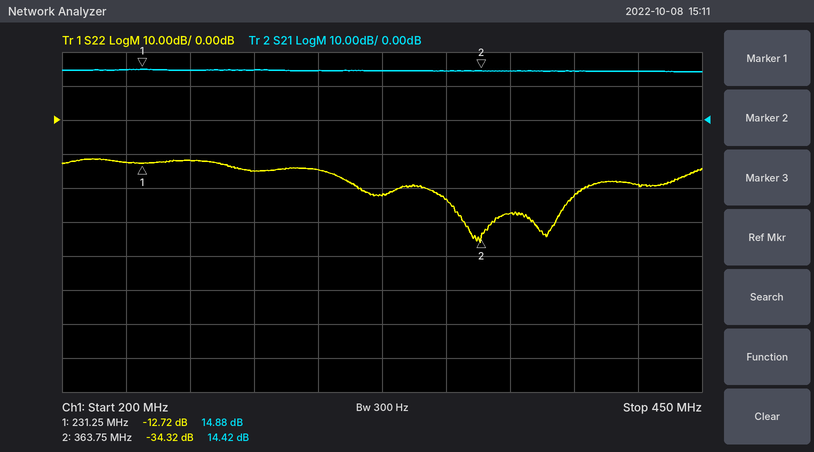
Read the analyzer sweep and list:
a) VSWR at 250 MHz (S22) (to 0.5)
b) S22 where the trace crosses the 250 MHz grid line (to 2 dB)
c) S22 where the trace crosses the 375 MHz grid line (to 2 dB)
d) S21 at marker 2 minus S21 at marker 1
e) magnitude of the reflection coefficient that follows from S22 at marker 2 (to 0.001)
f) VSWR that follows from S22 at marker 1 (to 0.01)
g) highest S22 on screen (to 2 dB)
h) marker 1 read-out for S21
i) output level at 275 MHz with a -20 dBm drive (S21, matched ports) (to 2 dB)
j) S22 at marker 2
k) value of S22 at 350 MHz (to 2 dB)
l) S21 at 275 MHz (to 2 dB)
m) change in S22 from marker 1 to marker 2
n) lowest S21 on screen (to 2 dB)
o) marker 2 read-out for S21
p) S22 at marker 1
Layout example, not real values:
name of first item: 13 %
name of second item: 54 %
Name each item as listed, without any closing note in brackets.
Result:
VSWR at 250 MHz (S22): 1.5
S22 where the trace crosses the 250 MHz grid line: -12 dB
S22 where the trace crosses the 375 MHz grid line: -28 dB
S21 at marker 2 minus S21 at marker 1: -0.46 dB
magnitude of the reflection coefficient that follows from S22 at marker 2: 0.019
VSWR that follows from S22 at marker 1: 1.60
highest S22 on screen: -12 dB
marker 1 read-out for S21: 14.88 dB
output level at 275 MHz with a -20 dBm drive (S21, matched ports): -6 dBm
S22 at marker 2: -34.32 dB
value of S22 at 350 MHz: -24 dB
S21 at 275 MHz: 14 dB
change in S22 from marker 1 to marker 2: -21.60 dB
lowest S21 on screen: 14 dB
marker 2 read-out for S21: 14.42 dB
S22 at marker 1: -12.72 dB
